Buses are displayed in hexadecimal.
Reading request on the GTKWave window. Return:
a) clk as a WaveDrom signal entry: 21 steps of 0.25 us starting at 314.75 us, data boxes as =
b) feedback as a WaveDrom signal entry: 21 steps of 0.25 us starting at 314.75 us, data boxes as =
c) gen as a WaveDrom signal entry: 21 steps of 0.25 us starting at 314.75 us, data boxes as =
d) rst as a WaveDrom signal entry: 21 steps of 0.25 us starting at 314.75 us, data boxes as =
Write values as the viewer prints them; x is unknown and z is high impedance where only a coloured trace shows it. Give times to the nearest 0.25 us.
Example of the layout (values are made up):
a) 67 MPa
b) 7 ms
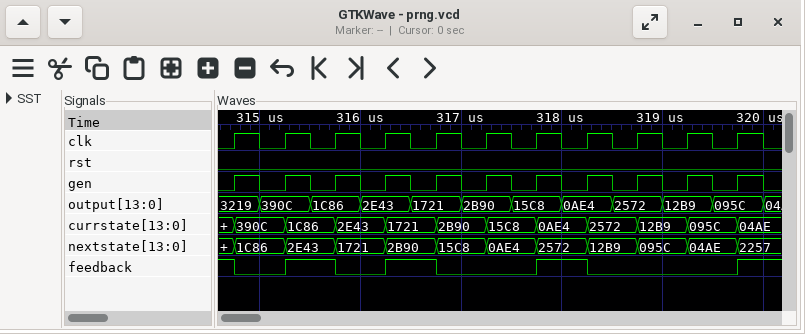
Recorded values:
a) {name: 'clk', wave: '101010101010101010101'}
b) {name: 'feedback', wave: '0.1.0.1.0...1.0.....1'}
c) {name: 'gen', wave: '101010101010101010101'}
d) {name: 'rst', wave: '0....................'}
